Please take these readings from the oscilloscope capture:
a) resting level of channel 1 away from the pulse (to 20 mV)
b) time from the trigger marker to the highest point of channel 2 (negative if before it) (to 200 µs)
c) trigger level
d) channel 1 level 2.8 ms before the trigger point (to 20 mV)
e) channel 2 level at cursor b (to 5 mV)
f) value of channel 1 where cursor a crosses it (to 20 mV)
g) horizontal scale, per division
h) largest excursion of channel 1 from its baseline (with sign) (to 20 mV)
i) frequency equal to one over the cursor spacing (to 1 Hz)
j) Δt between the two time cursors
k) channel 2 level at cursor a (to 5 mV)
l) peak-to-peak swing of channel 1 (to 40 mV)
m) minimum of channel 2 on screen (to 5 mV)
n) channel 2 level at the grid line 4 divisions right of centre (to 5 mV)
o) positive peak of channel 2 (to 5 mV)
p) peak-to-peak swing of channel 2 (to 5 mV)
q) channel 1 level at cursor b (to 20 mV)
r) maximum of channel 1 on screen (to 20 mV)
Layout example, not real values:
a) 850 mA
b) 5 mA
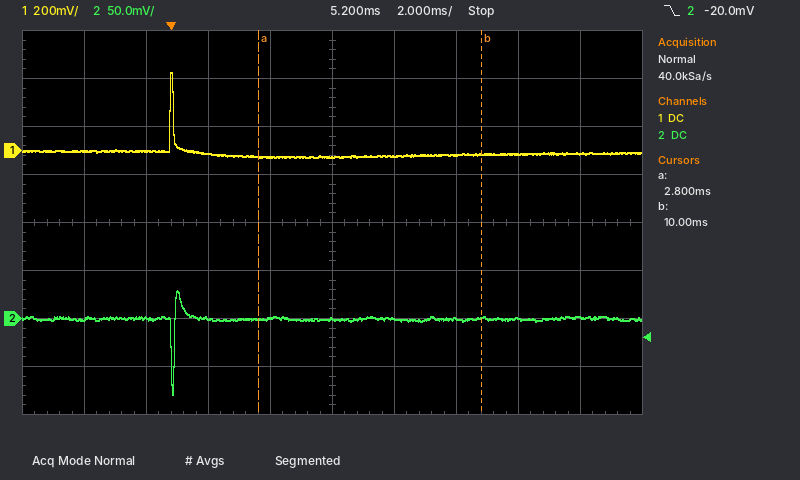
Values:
a) -20 mV
b) +200 µs
c) -20.0 mV
d) 0 mV
e) 0 mV
f) -20 mV
g) 2 ms
h) +340 mV
i) 139 Hz
j) 7.2 ms
k) 0 mV
l) 360 mV
m) -80 mV
n) 0 mV
o) 30 mV
p) 110 mV
q) -20 mV
r) 320 mV
